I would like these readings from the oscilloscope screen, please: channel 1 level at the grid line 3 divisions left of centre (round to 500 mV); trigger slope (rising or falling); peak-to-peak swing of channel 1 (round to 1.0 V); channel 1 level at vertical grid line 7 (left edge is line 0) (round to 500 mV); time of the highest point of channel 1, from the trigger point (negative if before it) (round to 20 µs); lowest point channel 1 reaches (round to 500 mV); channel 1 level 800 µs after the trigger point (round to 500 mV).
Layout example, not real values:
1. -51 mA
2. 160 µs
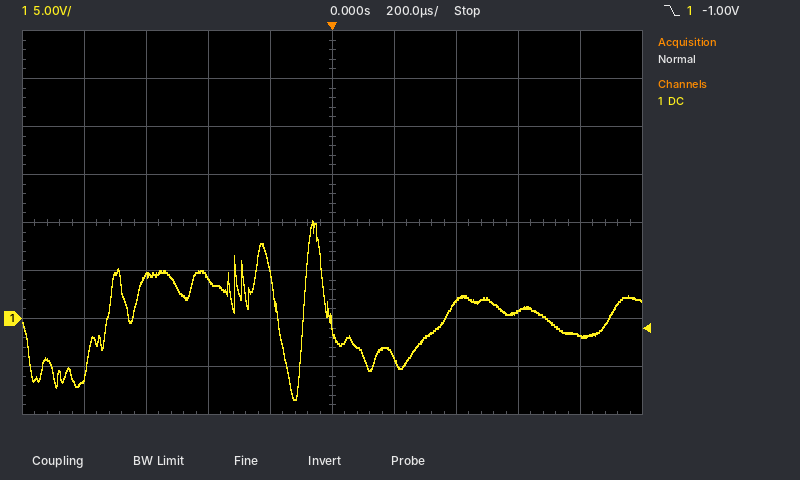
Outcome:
1. 4.5 V
2. falling
3. 19.0 V
4. 2.0 V
5. -60 µs
6. -8.5 V
7. -2.0 V
